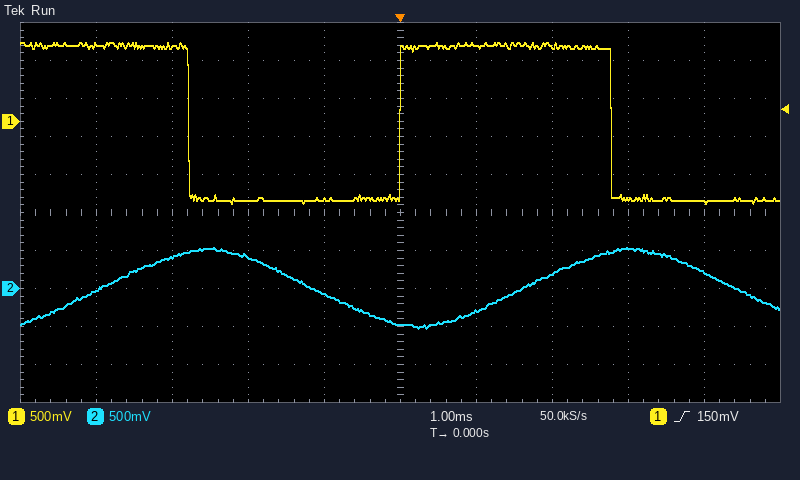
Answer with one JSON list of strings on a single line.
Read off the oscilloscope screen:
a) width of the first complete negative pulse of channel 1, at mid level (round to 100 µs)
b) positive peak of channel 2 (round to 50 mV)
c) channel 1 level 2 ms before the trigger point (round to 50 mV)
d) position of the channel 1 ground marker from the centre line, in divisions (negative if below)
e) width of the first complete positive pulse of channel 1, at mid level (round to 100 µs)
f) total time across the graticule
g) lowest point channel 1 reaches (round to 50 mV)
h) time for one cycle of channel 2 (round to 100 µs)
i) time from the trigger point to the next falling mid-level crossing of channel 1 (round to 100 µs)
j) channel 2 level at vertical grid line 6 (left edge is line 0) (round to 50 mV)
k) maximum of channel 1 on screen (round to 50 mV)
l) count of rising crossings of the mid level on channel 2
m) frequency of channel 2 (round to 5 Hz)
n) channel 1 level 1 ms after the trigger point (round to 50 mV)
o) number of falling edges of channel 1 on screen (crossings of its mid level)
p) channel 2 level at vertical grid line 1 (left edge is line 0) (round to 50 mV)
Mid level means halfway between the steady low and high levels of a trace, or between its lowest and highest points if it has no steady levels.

["2.8 ms", "550 mV", "-1.05 V", "+2.4 div", "2.8 ms", "10 ms", "-1.10 V", "5.6 ms", "2.8 ms", "-300 mV", "1.05 V", "2", "180 Hz", "1.00 V", "2", "0 mV"]
